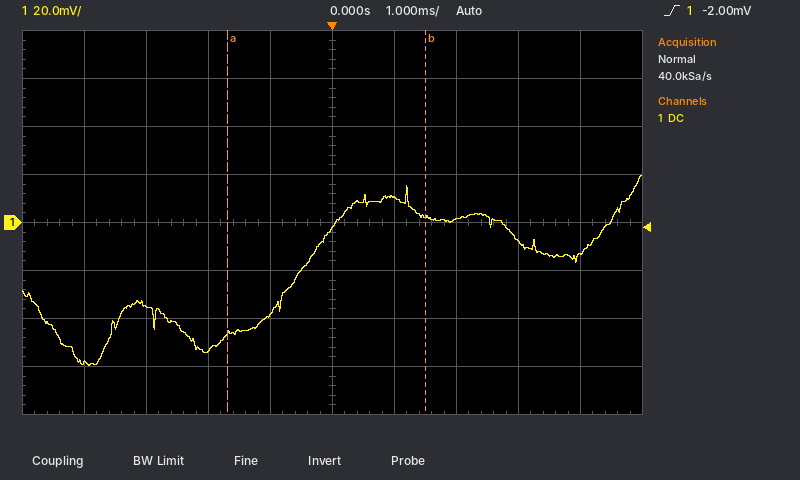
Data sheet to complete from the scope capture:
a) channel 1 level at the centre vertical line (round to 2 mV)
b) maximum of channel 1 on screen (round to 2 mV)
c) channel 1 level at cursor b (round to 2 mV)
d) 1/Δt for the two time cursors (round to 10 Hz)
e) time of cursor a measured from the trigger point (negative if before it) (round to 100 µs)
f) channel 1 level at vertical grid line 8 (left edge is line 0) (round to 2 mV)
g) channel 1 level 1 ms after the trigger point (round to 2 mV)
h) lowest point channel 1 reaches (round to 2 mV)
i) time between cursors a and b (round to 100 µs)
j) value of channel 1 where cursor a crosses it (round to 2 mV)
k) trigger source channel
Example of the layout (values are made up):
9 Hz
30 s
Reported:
-2 mV
20 mV
2 mV
310 Hz
-1.7 ms
-8 mV
10 mV
-60 mV
3.2 ms
-46 mV
channel 1
